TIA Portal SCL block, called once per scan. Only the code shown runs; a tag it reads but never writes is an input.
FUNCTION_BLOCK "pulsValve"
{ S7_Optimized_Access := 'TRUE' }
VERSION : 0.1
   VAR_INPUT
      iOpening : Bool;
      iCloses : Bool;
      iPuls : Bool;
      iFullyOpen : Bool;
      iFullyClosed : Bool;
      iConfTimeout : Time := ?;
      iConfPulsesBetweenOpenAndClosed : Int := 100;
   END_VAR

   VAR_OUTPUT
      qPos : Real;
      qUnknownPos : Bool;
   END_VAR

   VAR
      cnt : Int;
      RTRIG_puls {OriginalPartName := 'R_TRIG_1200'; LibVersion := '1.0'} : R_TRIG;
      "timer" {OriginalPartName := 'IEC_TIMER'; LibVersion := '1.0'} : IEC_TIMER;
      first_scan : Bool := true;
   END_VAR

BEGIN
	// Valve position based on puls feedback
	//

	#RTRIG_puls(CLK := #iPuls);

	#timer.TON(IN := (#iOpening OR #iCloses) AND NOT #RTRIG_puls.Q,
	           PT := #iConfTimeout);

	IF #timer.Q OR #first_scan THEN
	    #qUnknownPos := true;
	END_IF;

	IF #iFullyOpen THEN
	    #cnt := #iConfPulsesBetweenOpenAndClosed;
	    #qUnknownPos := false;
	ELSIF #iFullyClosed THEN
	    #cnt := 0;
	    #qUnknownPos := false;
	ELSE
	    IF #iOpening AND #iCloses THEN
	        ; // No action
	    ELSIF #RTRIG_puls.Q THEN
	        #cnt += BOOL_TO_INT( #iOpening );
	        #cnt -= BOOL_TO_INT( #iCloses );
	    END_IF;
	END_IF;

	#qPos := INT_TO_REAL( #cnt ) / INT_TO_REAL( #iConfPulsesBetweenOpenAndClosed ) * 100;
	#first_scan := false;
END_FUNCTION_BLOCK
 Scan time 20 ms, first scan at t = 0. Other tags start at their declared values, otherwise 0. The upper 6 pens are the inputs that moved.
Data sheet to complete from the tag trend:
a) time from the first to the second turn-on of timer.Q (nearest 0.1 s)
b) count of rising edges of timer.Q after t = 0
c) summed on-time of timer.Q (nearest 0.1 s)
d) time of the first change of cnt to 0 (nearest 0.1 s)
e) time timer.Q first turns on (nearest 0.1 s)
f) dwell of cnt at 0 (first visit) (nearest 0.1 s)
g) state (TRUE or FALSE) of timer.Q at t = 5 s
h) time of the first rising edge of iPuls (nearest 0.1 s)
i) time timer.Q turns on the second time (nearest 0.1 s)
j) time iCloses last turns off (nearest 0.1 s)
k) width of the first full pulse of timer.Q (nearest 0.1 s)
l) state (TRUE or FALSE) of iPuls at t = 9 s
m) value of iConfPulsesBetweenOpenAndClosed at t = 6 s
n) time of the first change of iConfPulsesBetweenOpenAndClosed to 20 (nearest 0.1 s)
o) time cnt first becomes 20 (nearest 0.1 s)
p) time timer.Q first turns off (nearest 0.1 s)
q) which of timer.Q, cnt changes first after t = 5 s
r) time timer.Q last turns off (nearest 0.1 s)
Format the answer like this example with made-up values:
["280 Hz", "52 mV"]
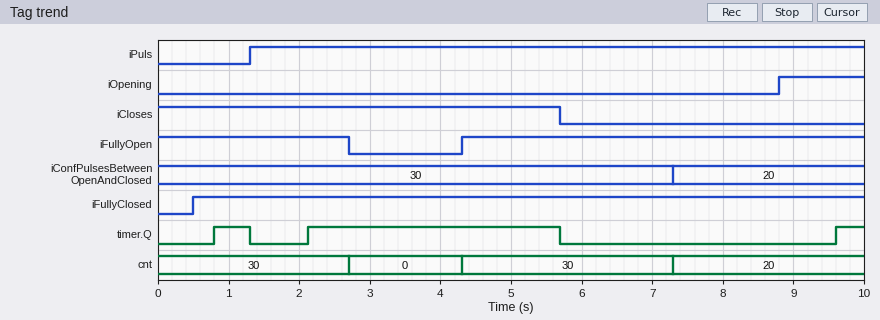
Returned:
["1.3 s", "3", "4.5 s", "2.7 s", "0.8 s", "1.6 s", "TRUE", "1.3 s", "2.1 s", "5.7 s", "0.5 s", "TRUE", "30", "7.3 s", "7.3 s", "1.3 s", "timer.Q", "5.7 s"]
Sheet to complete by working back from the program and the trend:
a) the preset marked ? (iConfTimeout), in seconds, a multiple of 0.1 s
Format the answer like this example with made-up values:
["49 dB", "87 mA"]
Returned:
["0.8 s"]
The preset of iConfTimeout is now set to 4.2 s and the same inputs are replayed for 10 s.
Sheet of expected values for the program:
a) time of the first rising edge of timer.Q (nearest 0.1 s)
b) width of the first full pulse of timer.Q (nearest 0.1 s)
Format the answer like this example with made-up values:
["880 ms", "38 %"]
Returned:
["5.5 s", "0.2 s"]
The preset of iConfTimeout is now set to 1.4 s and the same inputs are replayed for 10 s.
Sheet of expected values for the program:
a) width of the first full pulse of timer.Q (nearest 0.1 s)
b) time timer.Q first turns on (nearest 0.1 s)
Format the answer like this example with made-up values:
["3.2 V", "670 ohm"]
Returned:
["3.0 s", "2.7 s"]
